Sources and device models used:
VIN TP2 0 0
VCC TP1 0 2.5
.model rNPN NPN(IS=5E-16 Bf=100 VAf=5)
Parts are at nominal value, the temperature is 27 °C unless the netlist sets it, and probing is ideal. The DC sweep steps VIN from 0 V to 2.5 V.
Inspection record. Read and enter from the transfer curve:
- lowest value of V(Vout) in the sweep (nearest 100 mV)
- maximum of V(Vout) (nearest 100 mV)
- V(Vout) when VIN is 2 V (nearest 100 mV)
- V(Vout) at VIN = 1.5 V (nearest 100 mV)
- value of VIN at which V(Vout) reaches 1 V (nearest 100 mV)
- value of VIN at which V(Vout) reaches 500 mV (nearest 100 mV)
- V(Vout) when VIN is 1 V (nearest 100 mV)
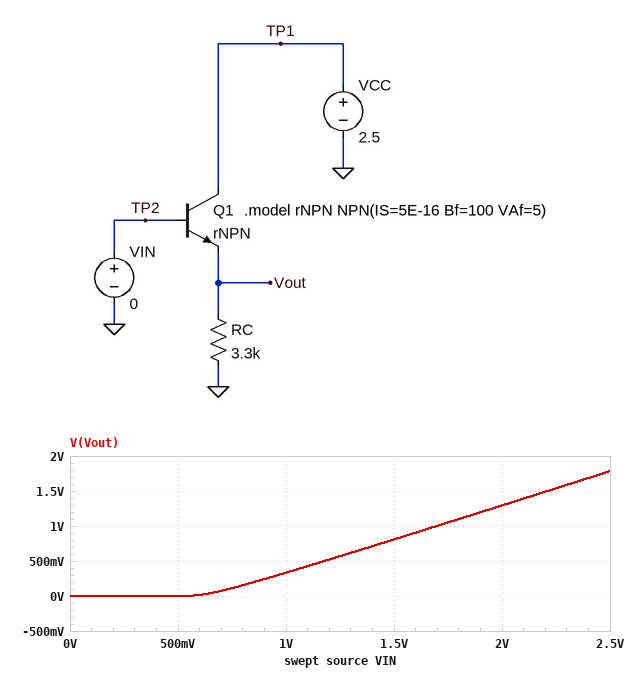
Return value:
0 V
1.8 V
1.3 V
800 mV
1.7 V
1.2 V
300 mV
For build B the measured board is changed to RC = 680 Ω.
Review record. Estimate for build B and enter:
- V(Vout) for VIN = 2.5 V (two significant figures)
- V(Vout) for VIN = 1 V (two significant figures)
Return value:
1.7 V
300 mV
